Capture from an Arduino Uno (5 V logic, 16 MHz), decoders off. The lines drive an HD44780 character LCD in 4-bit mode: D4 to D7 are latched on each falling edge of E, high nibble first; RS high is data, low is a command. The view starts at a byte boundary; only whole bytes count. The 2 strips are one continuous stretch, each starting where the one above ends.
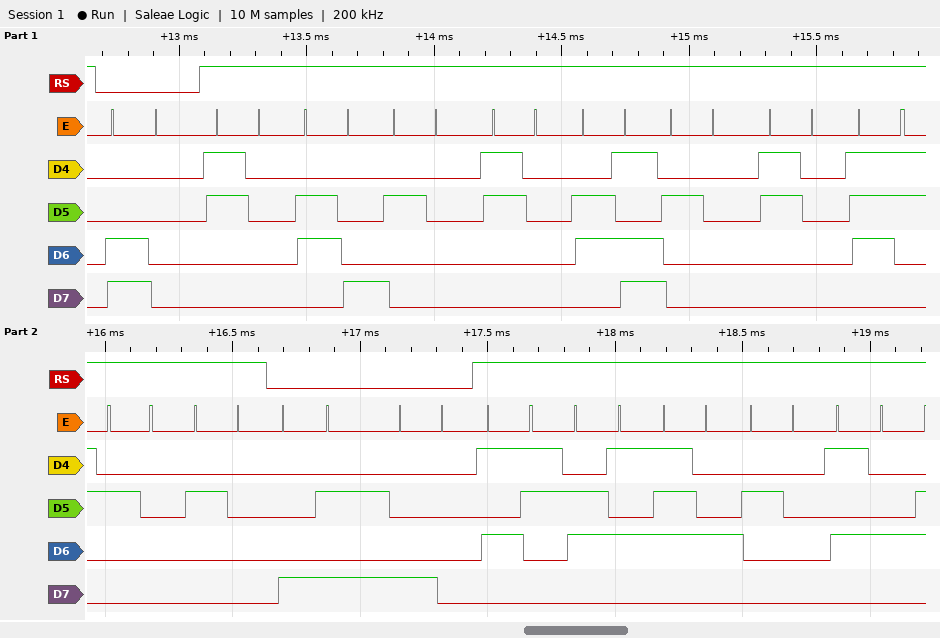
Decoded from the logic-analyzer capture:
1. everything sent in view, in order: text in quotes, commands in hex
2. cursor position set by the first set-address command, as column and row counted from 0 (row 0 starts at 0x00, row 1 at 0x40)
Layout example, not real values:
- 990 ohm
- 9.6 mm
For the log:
- 0xC0 "0h 0m 0s  " 0x8A 0x80 "Set T"
- column 0, row 1
